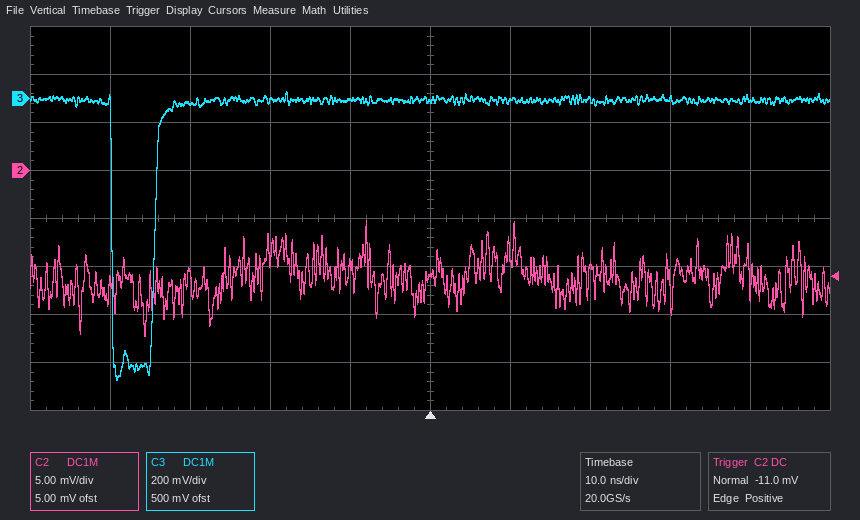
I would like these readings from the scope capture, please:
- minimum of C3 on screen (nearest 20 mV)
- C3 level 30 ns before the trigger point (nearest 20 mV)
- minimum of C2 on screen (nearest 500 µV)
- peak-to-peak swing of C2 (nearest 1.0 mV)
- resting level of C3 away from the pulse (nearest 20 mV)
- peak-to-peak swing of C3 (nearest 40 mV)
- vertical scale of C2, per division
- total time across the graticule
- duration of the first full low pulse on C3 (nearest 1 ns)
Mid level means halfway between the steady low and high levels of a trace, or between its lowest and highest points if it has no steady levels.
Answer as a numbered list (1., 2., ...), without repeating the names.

1. -1.18 V
2. -20 mV
3. -17.0 mV
4. 12.0 mV
5. 0 mV
6. 1.20 V
7. 5 mV
8. 100 ns
9. 5 ns
